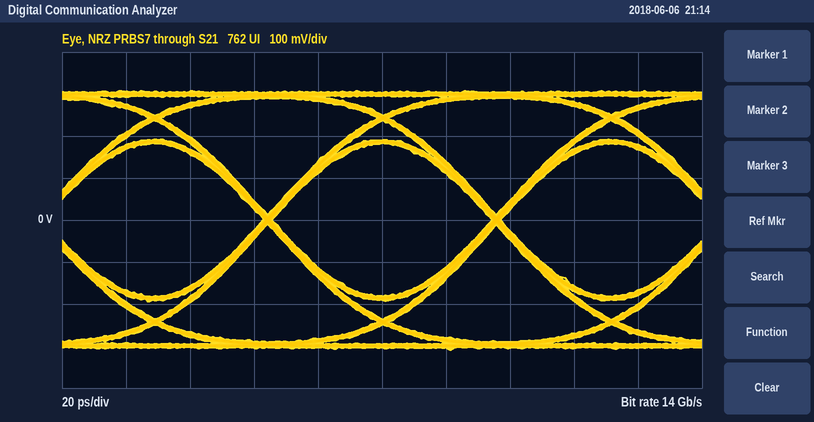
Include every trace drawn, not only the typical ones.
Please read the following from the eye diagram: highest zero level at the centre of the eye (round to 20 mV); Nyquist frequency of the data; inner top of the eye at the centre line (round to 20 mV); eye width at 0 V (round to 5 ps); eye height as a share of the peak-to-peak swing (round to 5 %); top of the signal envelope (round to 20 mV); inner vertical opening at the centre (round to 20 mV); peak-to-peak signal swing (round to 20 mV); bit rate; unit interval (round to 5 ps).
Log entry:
-180 mV
7 GHz
180 mV
70 ps
60 %
300 mV
360 mV
620 mV
14 Gb/s
70 ps
